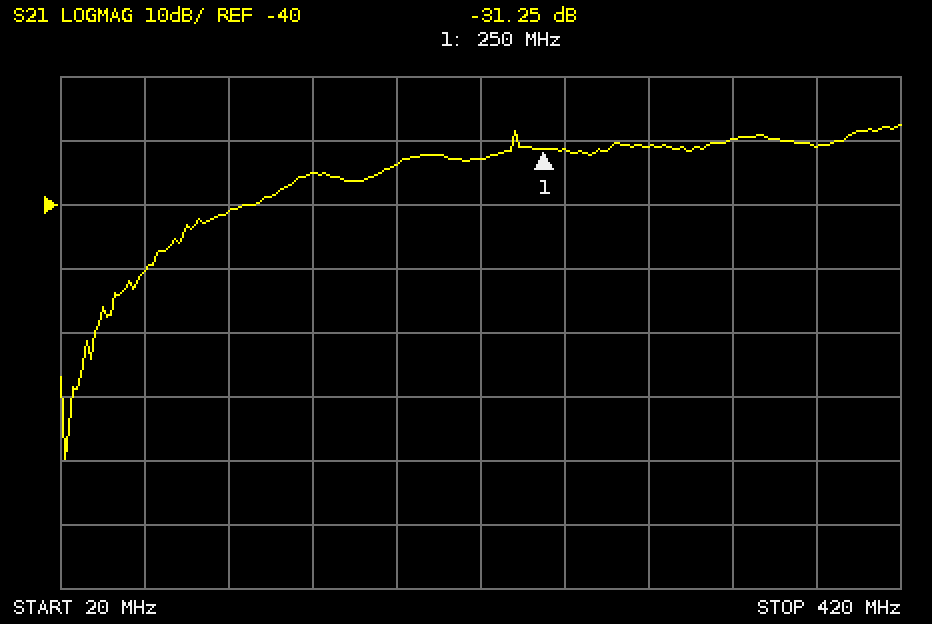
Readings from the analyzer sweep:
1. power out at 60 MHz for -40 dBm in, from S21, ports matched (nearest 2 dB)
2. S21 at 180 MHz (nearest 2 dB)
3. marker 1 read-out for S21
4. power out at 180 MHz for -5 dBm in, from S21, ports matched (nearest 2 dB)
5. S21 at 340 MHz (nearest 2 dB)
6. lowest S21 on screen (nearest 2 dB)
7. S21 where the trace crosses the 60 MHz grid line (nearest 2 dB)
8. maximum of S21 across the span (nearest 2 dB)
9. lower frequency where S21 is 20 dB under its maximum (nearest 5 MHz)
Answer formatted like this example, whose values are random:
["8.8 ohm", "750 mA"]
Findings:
["-90 dBm", "-34 dB", "-31.25 dB", "-38 dBm", "-30 dB", "-80 dB", "-50 dB", "-28 dB", "65 MHz"]
